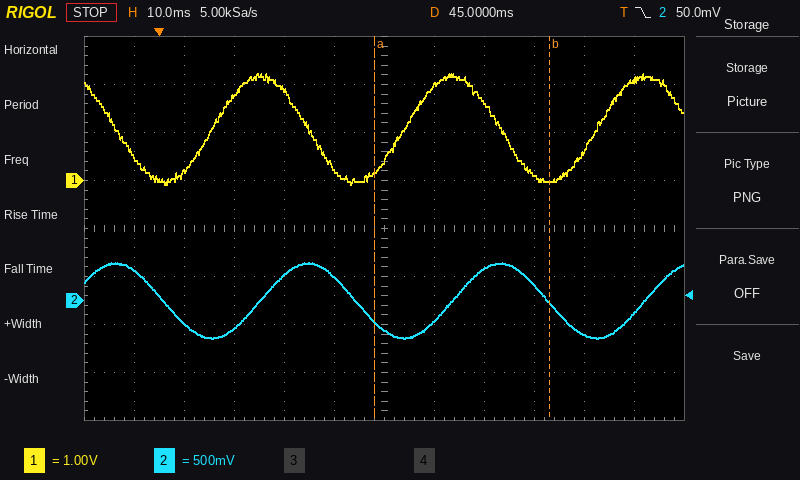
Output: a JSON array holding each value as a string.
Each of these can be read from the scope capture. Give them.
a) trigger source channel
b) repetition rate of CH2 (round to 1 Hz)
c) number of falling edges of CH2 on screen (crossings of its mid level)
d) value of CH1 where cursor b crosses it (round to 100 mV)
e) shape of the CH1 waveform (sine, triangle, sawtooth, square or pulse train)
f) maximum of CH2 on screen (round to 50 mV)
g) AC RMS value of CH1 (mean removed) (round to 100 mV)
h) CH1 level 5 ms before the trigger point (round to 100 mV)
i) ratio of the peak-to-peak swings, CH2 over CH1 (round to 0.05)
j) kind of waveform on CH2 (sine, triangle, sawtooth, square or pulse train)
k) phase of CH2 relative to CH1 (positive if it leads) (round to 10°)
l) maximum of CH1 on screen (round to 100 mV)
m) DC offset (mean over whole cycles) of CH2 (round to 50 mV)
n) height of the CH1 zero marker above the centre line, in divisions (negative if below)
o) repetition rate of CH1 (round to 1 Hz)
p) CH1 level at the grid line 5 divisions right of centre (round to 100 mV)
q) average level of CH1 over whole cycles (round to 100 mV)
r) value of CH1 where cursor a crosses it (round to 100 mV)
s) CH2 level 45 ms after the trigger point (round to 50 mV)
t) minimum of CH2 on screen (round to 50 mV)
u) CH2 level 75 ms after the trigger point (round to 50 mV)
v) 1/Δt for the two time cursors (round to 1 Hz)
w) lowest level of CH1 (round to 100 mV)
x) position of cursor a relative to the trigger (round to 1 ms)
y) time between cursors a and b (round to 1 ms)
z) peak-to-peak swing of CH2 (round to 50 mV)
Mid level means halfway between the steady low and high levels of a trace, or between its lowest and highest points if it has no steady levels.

["CH2", "26 Hz", "3", "0.0 V", "sine", "400 mV", "800 mV", "500 mV", "0.35", "sine", "-90°", "2.2 V", "0 mV", "+1.0 div", "26 Hz", "2.1 V", "1.1 V", "200 mV", "-300 mV", "-400 mV", "150 mV", "29 Hz", "-100 mV", "+43 ms", "35 ms", "800 mV"]
